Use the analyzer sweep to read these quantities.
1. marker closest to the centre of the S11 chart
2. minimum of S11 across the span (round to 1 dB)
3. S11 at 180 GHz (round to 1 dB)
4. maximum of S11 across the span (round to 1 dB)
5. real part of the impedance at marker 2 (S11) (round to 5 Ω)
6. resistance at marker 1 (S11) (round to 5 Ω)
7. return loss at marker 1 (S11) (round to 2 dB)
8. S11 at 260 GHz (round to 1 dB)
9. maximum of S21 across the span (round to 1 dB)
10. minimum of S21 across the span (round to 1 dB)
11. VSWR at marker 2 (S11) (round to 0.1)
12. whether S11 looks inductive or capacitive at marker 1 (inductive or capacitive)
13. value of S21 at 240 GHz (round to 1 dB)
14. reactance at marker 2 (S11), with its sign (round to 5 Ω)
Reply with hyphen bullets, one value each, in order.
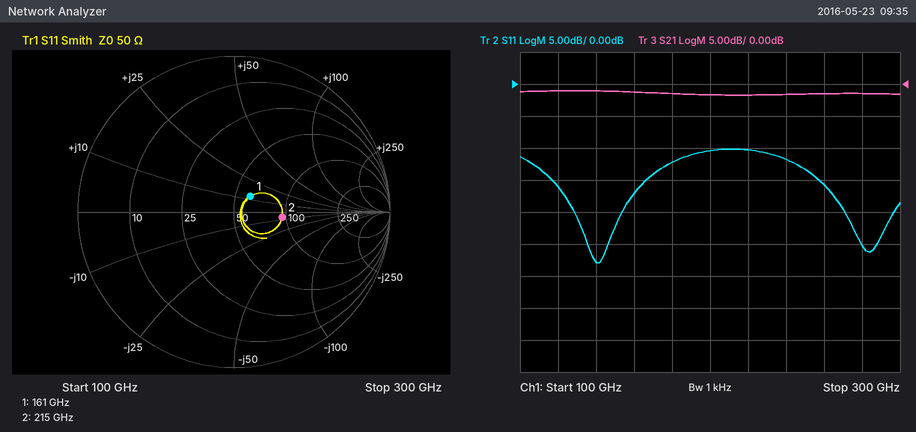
- marker 1
- -28 dB
- -12 dB
- -10 dB
- 95 Ω
- 60 Ω
- 16 dB
- -16 dB
- -1 dB
- -2 dB
- 1.9
- inductive
- -2 dB
- -5 Ω
